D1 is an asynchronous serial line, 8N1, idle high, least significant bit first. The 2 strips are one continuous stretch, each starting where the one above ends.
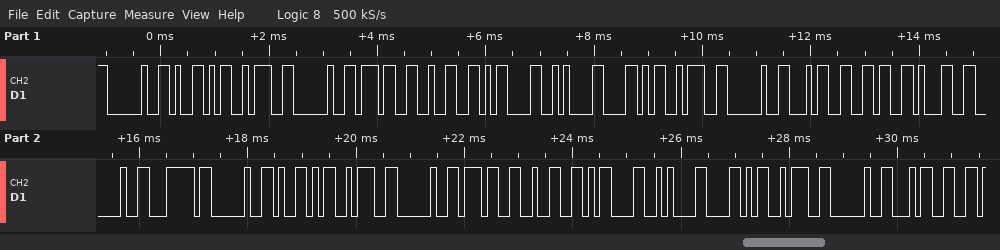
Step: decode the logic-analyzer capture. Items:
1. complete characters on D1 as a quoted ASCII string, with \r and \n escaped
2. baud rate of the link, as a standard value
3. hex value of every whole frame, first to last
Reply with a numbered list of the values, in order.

1. " Y: 72\r\nX: 461 | Y: 72\r\nX: 4"
2. 9600 baud
3. 20 59 3A 20 37 32 0D 0A 58 3A 20 34 36 31 20 7C 20 59 3A 20 37 32 0D 0A 58 3A 20 34
